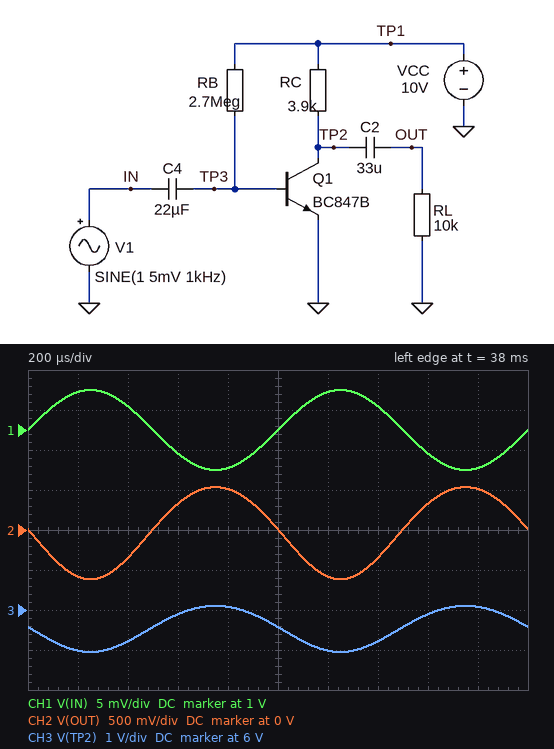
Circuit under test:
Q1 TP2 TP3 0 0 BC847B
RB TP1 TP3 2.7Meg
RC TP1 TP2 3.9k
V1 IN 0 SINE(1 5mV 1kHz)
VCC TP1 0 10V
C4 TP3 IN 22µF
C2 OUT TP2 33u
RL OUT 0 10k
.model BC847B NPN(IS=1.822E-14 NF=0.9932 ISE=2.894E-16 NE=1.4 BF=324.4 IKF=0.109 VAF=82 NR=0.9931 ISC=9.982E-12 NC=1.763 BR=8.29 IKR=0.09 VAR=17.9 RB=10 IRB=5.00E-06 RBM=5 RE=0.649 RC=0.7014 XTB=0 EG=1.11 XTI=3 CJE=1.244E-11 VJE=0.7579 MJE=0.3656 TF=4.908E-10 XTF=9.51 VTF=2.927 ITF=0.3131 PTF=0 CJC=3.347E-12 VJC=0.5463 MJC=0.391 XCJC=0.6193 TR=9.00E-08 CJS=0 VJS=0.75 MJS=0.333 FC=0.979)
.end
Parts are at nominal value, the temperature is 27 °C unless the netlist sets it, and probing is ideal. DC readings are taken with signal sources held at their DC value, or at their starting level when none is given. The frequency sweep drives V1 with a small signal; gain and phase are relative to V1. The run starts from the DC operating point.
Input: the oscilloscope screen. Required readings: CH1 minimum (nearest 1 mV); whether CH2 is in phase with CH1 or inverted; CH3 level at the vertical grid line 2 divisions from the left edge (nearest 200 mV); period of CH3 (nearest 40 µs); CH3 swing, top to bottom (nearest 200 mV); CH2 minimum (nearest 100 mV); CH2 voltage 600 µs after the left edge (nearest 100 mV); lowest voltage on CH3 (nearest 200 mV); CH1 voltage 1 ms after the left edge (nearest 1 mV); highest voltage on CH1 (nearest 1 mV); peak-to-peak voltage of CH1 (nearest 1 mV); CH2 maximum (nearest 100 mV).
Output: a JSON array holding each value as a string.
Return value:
["995 mV", "inverted", "5.2 V", "1.00 ms", "1.2 V", "-600 mV", "300 mV", "5.0 V", "1.000 V", "1.005 V", "10 mV", "500 mV"]
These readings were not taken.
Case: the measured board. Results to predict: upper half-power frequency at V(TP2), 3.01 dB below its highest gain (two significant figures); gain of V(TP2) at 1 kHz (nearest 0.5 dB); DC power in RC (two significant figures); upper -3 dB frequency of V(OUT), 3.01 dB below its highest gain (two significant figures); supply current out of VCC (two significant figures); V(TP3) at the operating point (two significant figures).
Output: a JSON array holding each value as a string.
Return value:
["35 MHz", "41.0 dB", "5.0 mW", "35 MHz", "1.1 mA", "640 mV"]
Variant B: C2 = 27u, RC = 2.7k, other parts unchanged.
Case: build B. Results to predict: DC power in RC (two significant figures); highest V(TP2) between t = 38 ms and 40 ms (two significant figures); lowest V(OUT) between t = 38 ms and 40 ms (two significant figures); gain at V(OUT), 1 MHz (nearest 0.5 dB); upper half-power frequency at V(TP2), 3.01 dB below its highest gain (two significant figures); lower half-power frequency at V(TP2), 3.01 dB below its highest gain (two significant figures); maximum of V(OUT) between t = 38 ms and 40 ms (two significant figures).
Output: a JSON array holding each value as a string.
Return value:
["3.6 mW", "7.3 V", "-480 mV", "39.0 dB", "49 MHz", "840 mHz", "420 mV"]
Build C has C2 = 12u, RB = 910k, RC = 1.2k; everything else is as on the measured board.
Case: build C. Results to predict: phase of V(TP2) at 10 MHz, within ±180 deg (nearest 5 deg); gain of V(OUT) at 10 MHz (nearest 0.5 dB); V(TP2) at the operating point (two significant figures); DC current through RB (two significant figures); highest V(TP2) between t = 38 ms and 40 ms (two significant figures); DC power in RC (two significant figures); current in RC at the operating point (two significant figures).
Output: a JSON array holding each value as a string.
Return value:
["170 deg", "41.5 dB", "6.0 V", "10 µA", "6.6 V", "13 mW", "3.3 mA"]
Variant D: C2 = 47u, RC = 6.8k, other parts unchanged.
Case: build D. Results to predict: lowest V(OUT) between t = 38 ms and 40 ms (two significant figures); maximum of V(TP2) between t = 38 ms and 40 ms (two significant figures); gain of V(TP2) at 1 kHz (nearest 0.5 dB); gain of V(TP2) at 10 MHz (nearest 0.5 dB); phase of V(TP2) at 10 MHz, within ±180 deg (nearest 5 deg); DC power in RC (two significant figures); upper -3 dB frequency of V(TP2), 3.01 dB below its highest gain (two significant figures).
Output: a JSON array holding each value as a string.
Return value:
["-840 mV", "3.3 V", "44.0 dB", "43.0 dB", "150 deg", "8.2 mW", "18 MHz"]
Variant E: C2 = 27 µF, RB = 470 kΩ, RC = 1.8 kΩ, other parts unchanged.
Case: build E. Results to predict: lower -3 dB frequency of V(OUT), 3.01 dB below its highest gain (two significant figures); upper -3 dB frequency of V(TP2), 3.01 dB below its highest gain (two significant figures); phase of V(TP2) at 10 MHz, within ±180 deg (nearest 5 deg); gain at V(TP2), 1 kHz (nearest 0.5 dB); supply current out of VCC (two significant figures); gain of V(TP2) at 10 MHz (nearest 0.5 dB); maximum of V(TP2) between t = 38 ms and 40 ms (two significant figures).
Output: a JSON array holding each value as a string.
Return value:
["55 Hz", "2.7 MHz", "105 deg", "45.0 dB", "5.5 mA", "33.5 dB", "2.1 V"]
